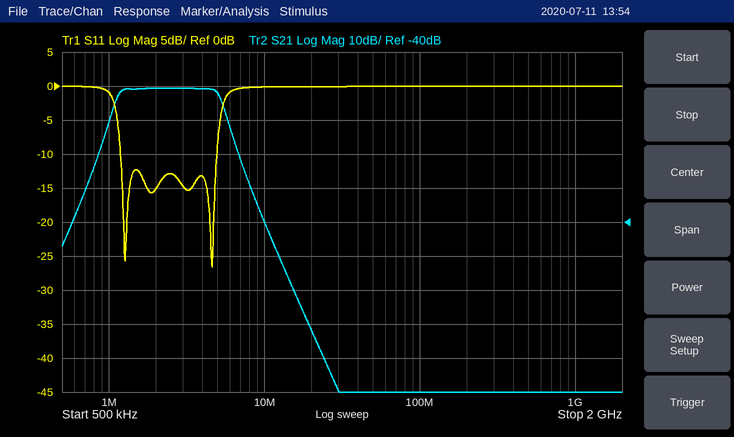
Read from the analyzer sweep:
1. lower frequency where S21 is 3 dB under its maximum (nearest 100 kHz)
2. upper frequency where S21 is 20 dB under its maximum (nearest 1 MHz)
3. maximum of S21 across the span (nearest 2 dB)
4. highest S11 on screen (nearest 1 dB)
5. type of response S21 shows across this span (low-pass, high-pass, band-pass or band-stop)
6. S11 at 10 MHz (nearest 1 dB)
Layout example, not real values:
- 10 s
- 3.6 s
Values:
- 1.1 MHz
- 7 MHz
- 0 dB
- 0 dB
- band-pass
- 0 dB
